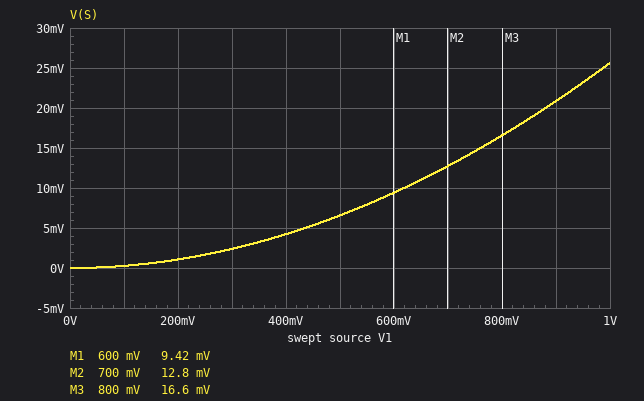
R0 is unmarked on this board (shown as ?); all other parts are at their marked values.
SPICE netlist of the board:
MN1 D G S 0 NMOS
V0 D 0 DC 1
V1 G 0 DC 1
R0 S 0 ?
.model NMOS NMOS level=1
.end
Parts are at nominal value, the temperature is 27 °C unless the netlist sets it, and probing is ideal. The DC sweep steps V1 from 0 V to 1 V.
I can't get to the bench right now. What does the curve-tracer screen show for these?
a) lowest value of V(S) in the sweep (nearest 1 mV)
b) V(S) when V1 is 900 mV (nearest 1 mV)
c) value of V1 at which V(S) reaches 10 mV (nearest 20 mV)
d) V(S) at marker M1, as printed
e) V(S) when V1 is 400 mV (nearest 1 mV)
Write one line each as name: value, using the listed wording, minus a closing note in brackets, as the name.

lowest value of V(S) in the sweep: 0 V
V(S) when V1 is 900 mV: 21 mV
value of V1 at which V(S) reaches 10 mV: 620 mV
V(S) at marker M1, as printed: 9.42 mV
V(S) when V1 is 400 mV: 4 mV
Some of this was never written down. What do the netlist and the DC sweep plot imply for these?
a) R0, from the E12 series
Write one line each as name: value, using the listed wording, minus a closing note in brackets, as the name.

R0, from the E12 series: 2.7 kΩ
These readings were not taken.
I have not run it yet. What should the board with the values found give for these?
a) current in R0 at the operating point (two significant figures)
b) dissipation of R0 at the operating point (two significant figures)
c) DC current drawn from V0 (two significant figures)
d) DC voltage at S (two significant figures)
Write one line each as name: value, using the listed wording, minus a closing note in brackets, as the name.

current in R0 at the operating point: 9.5 µA
dissipation of R0 at the operating point: 240 nW
DC current drawn from V0: 9.5 µA
DC voltage at S: 26 mV
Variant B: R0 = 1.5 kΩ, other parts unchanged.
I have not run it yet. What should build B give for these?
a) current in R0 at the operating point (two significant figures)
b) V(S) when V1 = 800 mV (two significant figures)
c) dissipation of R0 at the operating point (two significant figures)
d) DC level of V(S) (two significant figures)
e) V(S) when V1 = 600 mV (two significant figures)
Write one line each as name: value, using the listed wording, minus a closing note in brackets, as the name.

current in R0 at the operating point: 9.7 µA
V(S) when V1 = 800 mV: 9.4 mV
dissipation of R0 at the operating point: 140 nW
DC level of V(S): 15 mV
V(S) when V1 = 600 mV: 5.3 mV
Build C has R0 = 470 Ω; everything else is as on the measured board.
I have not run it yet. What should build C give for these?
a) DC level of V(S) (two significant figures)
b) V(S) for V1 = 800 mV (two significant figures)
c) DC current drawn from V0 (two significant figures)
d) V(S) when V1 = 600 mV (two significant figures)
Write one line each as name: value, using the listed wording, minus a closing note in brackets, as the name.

DC level of V(S): 4.7 mV
V(S) for V1 = 800 mV: 3.0 mV
DC current drawn from V0: 9.9 µA
V(S) when V1 = 600 mV: 1.7 mV
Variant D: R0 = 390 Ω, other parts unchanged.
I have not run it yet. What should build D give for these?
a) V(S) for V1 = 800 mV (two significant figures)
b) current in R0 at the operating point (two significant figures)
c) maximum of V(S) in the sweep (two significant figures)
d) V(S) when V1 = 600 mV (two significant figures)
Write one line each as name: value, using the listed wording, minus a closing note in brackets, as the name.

V(S) for V1 = 800 mV: 2.5 mV
current in R0 at the operating point: 9.9 µA
maximum of V(S) in the sweep: 3.9 mV
V(S) when V1 = 600 mV: 1.4 mV
